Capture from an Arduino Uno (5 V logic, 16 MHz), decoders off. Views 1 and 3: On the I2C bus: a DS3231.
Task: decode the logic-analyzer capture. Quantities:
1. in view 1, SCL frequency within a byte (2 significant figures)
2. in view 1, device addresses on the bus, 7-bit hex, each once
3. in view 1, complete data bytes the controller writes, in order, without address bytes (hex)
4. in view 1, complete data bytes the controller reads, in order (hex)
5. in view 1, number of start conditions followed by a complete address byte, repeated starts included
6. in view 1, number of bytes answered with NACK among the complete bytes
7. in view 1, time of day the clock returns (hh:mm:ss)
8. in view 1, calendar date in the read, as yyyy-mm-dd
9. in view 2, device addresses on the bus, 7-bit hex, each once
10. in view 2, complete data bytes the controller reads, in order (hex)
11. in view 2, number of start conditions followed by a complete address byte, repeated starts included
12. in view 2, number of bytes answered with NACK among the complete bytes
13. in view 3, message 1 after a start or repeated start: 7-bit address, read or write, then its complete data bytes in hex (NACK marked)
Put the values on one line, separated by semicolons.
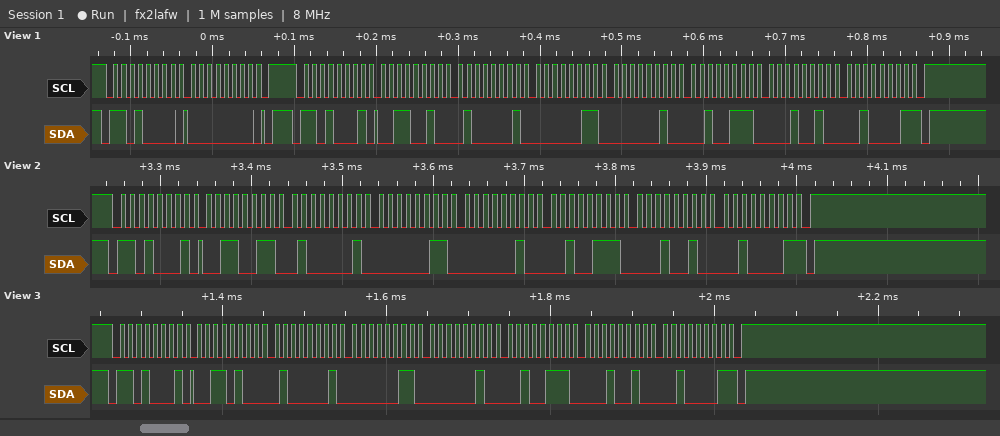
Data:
100 kHz; 0x68; 00; 32 41 03 02 27 12 21; 2; 1; 03:41:32; 2021-12-27; 0x68; 33 41 03 02 27 12 21; 1; 1; 0x68 read: 34 41 03 02 27 12 21 NACK
